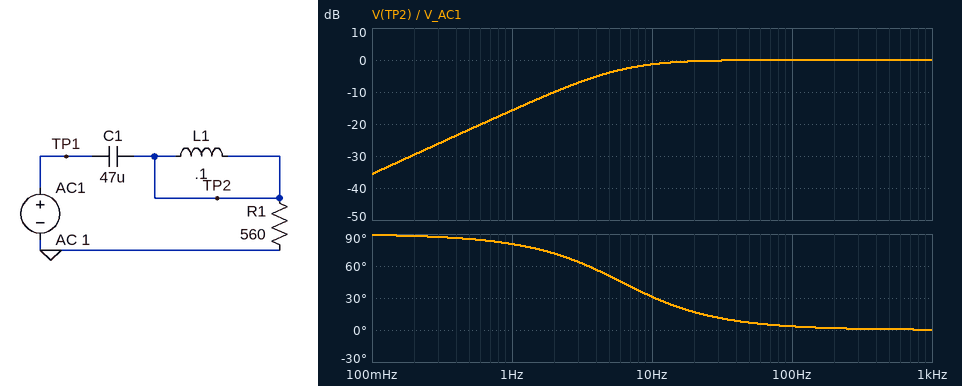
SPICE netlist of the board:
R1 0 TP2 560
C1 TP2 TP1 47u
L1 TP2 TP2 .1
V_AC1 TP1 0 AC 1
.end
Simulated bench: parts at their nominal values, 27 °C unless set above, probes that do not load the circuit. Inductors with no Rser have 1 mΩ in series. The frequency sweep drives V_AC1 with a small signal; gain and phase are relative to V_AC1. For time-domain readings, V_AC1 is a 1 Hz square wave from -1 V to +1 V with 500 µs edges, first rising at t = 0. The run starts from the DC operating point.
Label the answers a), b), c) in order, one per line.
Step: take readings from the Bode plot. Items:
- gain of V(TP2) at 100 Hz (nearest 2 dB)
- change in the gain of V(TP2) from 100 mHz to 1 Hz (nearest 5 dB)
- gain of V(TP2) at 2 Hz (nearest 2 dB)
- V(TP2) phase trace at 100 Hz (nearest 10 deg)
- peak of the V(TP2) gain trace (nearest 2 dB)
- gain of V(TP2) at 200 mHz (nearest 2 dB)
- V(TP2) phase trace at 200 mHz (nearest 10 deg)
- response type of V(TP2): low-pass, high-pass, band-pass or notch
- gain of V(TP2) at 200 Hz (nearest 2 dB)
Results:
a) 0 dB
b) 20 dB
c) -10 dB
d) 0 deg
e) 0 dB
f) -30 dB
g) 90 deg
h) high-pass
i) 0 dB
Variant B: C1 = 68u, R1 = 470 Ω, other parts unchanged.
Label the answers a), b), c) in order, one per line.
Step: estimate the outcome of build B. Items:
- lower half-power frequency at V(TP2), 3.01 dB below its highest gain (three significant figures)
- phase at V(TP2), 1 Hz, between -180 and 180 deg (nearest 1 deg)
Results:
a) 4.98 Hz
b) 79 deg
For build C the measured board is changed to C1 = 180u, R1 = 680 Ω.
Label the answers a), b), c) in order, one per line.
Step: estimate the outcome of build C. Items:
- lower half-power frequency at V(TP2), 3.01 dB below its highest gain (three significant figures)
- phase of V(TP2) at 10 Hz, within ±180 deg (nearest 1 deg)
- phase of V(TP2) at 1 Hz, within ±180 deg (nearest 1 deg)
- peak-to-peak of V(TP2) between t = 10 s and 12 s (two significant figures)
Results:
a) 1.30 Hz
b) 7 deg
c) 52 deg
d) 3.9 V
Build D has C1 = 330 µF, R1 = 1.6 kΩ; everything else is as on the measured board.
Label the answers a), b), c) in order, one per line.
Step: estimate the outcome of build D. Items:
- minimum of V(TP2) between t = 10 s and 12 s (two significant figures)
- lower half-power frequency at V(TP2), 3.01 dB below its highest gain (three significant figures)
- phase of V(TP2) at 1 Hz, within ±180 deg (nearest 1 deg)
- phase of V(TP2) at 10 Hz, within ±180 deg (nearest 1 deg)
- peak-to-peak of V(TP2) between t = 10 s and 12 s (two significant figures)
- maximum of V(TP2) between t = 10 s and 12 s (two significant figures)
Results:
a) -1.4 V
b) 301 mHz
c) 17 deg
d) 2 deg
e) 2.9 V
f) 1.4 V
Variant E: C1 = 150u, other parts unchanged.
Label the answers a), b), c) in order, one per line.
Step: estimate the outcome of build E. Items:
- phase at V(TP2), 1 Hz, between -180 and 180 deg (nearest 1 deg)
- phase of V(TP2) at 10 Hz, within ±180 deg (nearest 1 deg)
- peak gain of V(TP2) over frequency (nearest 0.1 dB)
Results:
a) 62 deg
b) 11 deg
c) 0 dB
